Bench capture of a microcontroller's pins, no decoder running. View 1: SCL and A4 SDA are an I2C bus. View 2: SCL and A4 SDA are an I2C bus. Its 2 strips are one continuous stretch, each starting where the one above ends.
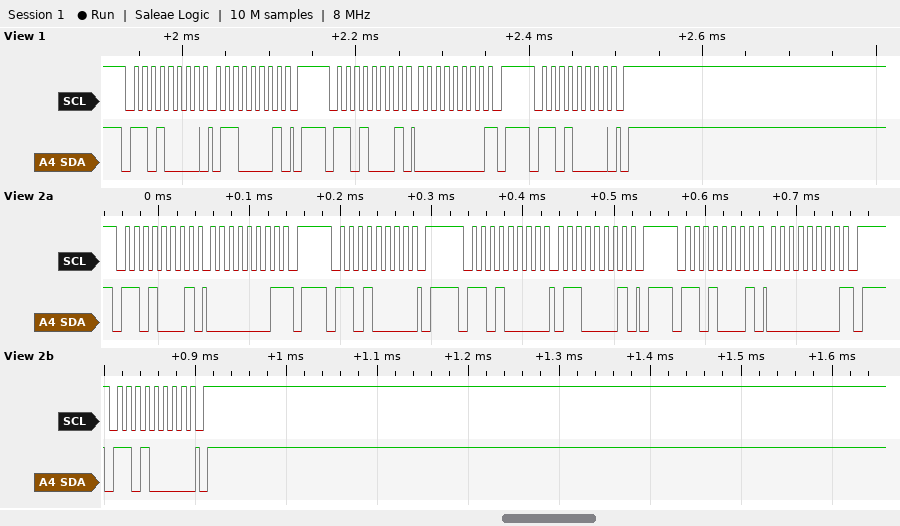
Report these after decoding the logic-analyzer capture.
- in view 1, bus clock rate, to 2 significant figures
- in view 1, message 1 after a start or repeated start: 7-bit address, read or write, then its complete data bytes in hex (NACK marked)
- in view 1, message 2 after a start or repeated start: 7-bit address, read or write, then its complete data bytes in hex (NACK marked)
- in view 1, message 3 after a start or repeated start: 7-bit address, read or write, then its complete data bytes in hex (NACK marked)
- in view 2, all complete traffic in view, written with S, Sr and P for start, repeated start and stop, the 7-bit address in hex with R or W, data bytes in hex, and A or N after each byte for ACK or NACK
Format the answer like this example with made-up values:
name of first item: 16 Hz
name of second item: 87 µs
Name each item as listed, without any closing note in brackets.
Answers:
in view 1, bus clock rate, to 2 significant figures: 100 kHz
in view 1, message 1 after a start or repeated start: 7-bit address, read or write, then its complete data bytes in hex: 0x68 write: 61
in view 1, message 2 after a start or repeated start: 7-bit address, read or write, then its complete data bytes in hex: 0x68 read: 00 NACK
in view 1, message 3 after a start or repeated start: 7-bit address, read or write, then its complete data bytes in hex: 0x68 write
in view 2, all complete traffic in view, written with S, Sr and P for start, repeated start and stop, the 7-bit address in hex with R or W, data bytes in hex, and A or N after each byte for ACK or NACK: S 68R A 01 N P S 68W A P S 68W A 61 A P S 68R A 00 N P S 68W A P
